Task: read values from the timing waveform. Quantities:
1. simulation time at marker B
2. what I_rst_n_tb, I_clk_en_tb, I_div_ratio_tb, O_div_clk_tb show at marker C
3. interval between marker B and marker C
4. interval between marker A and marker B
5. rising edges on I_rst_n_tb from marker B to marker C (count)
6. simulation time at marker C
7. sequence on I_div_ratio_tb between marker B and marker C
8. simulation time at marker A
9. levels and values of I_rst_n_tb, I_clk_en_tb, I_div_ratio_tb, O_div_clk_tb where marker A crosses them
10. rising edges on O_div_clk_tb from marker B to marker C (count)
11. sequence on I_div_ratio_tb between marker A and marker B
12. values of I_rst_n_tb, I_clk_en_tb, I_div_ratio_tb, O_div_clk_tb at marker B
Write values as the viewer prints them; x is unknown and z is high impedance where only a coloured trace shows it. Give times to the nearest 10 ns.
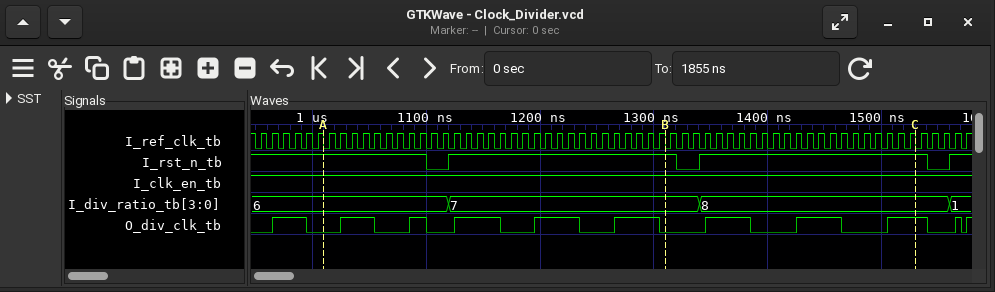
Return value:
1310 ns
I_rst_n_tb=1, I_clk_en_tb=1, I_div_ratio_tb=8, O_div_clk_tb=1
220 ns
300 ns
1
1530 ns
7, 8
1010 ns
I_rst_n_tb=1, I_clk_en_tb=1, I_div_ratio_tb=6, O_div_clk_tb=0
3
6, 7
I_rst_n_tb=1, I_clk_en_tb=1, I_div_ratio_tb=7, O_div_clk_tb=0
